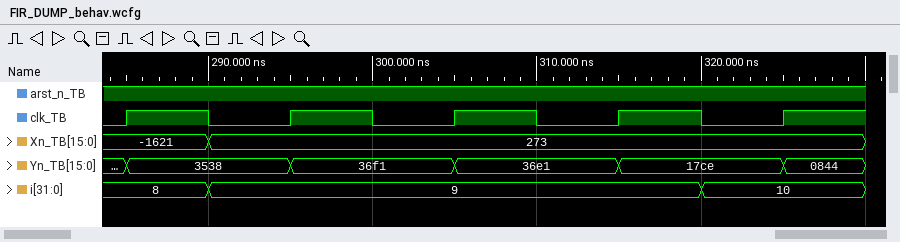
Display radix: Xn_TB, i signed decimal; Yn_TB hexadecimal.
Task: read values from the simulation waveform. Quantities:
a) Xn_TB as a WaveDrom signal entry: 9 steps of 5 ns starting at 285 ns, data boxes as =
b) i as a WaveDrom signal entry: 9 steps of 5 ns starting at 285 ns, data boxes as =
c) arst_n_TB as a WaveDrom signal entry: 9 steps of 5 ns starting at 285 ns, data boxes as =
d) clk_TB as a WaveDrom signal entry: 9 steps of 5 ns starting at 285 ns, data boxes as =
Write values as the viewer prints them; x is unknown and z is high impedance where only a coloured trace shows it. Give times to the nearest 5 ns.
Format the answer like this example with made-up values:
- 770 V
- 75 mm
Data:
- {name: 'Xn_TB', wave: '==.......', data: '-1621 273'}
- {name: 'i', wave: '==.....=.', data: '8 9 10'}
- {name: 'arst_n_TB', wave: '1........'}
- {name: 'clk_TB', wave: '101010101'}
